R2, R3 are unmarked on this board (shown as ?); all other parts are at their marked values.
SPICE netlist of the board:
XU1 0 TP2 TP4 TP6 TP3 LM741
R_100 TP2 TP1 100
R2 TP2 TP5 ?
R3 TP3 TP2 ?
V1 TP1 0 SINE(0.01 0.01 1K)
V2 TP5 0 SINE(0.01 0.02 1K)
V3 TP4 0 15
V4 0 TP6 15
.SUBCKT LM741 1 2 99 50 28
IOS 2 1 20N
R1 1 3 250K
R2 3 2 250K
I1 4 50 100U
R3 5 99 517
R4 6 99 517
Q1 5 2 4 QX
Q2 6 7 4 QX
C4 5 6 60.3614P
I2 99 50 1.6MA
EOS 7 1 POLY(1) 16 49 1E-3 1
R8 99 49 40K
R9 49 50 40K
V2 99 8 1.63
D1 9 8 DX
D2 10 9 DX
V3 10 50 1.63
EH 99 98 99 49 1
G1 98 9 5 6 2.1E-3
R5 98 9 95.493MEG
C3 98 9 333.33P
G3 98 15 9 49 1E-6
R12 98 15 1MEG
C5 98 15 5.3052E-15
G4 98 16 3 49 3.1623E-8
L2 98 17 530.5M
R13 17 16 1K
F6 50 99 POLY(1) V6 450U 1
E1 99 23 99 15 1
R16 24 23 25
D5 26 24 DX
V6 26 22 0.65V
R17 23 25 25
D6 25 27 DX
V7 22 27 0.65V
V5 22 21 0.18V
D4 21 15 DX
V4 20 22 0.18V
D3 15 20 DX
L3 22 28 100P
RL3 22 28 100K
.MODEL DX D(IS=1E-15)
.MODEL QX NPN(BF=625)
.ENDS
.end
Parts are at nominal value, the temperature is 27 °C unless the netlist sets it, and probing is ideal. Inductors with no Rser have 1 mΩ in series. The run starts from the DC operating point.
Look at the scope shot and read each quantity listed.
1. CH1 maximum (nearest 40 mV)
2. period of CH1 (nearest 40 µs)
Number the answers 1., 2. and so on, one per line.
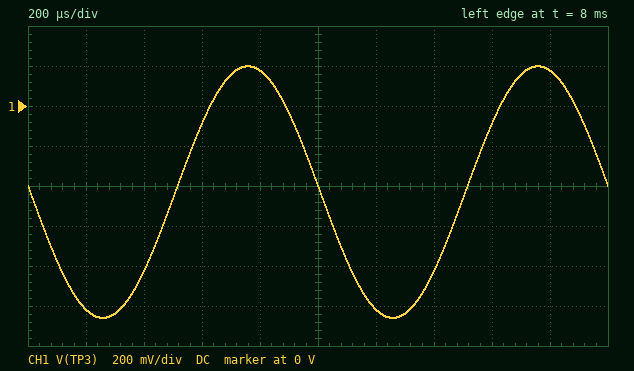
1. 200 mV
2. 1.00 ms
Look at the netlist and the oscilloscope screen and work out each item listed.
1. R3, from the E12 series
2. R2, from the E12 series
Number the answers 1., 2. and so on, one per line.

1. 3.3 kΩ
2. 220 Ω
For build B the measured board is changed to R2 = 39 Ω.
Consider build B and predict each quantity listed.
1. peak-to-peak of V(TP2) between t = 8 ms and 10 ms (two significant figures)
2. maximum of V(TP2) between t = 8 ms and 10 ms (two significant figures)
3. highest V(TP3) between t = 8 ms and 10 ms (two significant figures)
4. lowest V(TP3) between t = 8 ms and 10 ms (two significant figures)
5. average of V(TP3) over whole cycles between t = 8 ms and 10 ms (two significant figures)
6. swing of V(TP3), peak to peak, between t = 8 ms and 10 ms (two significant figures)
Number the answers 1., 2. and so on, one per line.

1. 4.1 mV
2. 3.1 mV
3. 950 mV
4. -3.1 V
5. -1.1 V
6. 4.0 V
